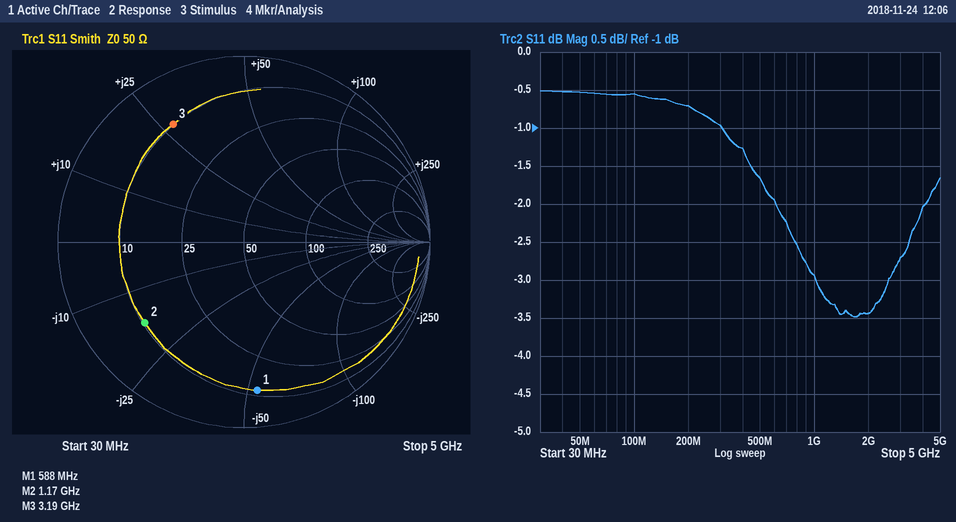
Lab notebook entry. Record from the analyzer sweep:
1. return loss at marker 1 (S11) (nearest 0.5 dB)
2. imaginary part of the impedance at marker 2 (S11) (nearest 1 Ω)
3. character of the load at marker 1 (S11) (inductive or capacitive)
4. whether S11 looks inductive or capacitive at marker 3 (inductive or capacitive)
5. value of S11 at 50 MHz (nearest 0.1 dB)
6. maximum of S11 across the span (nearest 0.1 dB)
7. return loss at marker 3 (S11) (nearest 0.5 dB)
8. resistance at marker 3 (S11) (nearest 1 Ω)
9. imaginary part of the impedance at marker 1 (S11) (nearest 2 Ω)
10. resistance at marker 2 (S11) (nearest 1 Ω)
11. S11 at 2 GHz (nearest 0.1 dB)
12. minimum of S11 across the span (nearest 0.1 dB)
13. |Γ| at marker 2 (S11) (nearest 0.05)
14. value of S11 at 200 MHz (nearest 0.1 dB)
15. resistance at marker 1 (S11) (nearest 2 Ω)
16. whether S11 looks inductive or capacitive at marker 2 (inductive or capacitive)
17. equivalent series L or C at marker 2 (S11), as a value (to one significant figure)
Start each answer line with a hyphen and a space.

- 2.0 dB
- -17 Ω
- capacitive
- inductive
- -0.5 dB
- -0.5 dB
- 2.5 dB
- 10 Ω
- -54 Ω
- 10 Ω
- -3.4 dB
- -3.5 dB
- 0.70
- -0.7 dB
- 12 Ω
- capacitive
- 8 pF
